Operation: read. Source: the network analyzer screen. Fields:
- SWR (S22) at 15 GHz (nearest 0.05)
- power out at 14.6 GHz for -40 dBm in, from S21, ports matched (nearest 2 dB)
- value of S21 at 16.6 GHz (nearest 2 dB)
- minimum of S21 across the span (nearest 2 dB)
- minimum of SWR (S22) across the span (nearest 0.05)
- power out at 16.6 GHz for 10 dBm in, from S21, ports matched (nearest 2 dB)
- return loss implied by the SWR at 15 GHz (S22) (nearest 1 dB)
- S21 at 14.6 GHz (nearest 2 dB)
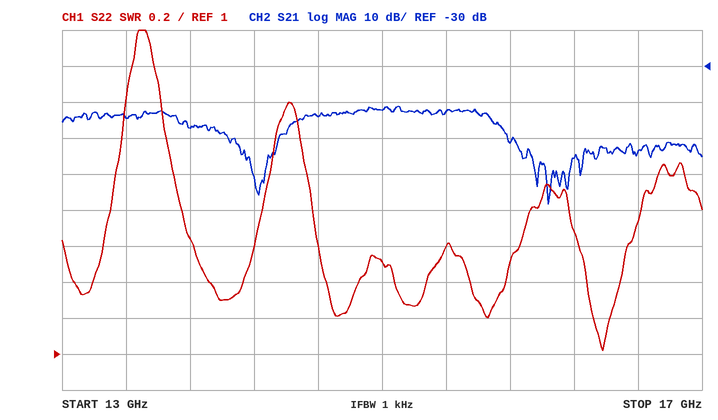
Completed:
1.50
-84 dBm
-54 dB
-68 dB
1.00
-44 dBm
14 dB
-44 dB
